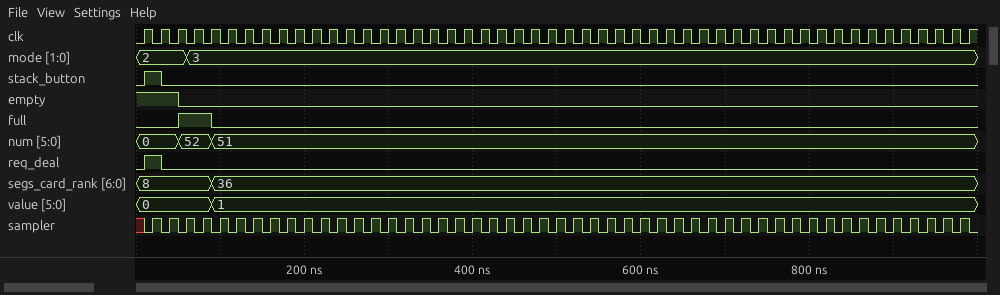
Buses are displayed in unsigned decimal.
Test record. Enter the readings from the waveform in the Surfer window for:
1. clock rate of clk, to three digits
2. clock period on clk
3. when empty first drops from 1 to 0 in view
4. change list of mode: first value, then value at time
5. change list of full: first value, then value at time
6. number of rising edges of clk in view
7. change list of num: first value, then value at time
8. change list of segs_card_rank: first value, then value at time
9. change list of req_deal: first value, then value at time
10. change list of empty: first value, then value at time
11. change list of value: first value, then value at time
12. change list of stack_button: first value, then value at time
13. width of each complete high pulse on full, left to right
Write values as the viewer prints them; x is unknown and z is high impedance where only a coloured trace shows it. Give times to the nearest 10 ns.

50.0 MHz
20 ns
50 ns
2, 3 at 60 ns
0, 1 at 50 ns, 0 at 90 ns
50
0, 52 at 50 ns, 51 at 90 ns
8, 36 at 90 ns
0, 1 at 10 ns, 0 at 30 ns
1, 0 at 50 ns
0, 1 at 90 ns
0, 1 at 10 ns, 0 at 30 ns
40 ns
